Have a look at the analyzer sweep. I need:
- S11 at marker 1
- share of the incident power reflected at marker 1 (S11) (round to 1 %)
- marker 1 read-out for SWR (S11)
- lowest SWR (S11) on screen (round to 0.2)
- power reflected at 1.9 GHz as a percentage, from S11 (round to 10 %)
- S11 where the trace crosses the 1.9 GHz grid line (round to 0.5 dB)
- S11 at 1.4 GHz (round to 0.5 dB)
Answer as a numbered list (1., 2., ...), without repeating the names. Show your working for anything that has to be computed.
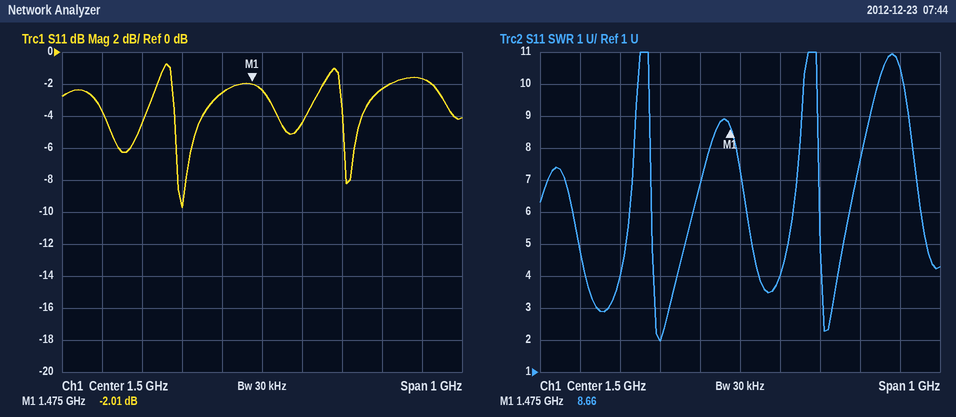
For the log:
1. -2.01 dB
2. 10^(-2.01/10) ≈ 63 %
3. 8.66
4. 2.0
5. 10^(-1.5/10) ≈ 70.8 %, so 70 % to the nearest 10 %
6. -1.5 dB
7. -2.5 dB
